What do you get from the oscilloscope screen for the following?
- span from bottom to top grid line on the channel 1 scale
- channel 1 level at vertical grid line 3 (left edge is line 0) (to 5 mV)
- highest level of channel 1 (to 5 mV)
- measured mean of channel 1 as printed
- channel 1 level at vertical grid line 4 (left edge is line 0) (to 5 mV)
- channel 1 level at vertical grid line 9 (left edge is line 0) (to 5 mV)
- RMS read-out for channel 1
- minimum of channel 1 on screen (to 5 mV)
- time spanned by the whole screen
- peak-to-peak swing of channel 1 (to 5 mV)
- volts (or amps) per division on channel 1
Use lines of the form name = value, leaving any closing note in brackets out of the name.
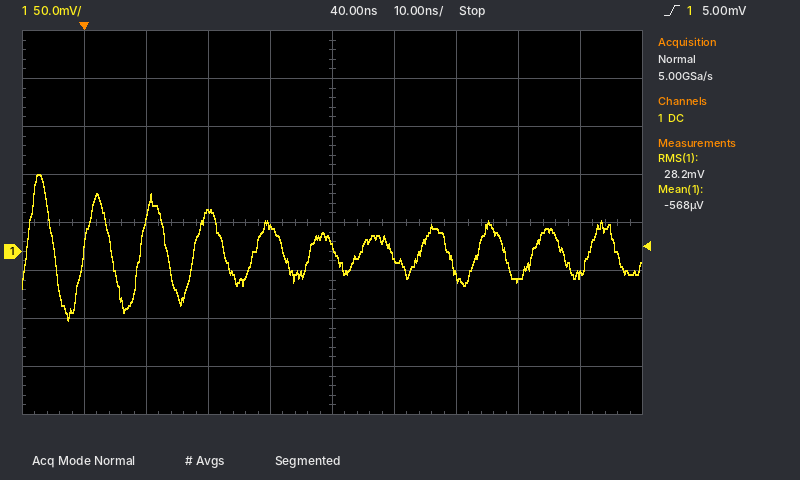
span from bottom to top grid line on the channel 1 scale = 400 mV
channel 1 level at vertical grid line 3 (left edge is line 0) = 40 mV
highest level of channel 1 = 80 mV
measured mean of channel 1 as printed = -568 µV
channel 1 level at vertical grid line 4 (left edge is line 0) = 30 mV
channel 1 level at vertical grid line 9 (left edge is line 0) = -25 mV
RMS read-out for channel 1 = 28.2 mV
minimum of channel 1 on screen = -70 mV
time spanned by the whole screen = 100 ns
peak-to-peak swing of channel 1 = 150 mV
volts (or amps) per division on channel 1 = 50 mV
